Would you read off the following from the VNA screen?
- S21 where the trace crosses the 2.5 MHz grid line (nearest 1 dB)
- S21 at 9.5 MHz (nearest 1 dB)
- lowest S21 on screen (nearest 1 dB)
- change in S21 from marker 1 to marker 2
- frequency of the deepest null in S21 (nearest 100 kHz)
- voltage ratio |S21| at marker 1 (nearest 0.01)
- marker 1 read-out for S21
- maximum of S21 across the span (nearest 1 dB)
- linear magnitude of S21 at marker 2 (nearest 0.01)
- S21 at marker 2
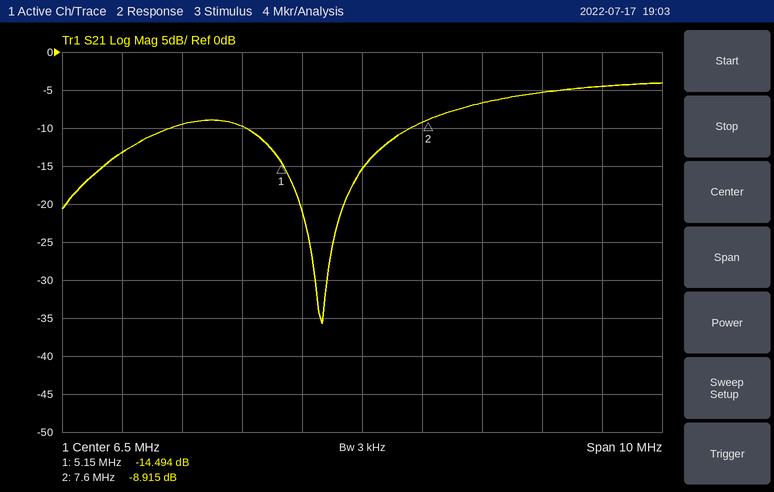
-13 dB
-5 dB
-36 dB
5.579 dB
5.8 MHz
0.19
-14.494 dB
-4 dB
0.36
-8.915 dB
